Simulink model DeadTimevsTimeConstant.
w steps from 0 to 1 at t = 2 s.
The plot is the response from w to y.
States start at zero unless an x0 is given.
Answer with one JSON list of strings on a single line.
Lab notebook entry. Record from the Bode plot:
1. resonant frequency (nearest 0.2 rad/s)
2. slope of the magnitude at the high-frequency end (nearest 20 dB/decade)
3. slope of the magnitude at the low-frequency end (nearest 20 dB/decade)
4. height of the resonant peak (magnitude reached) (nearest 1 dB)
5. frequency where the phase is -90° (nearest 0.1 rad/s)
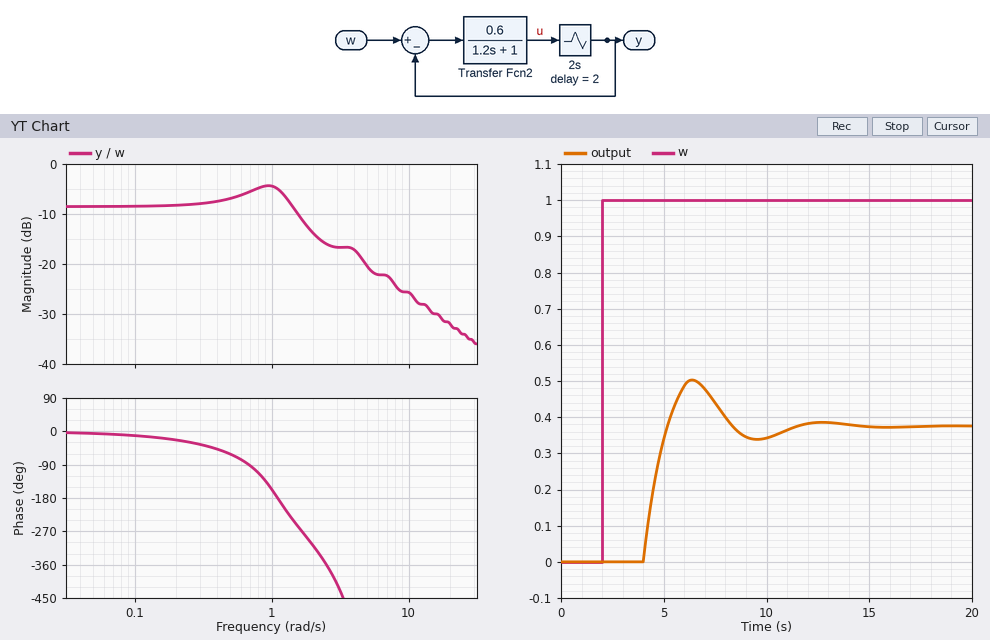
["1.0 rad/s", "-20 dB/decade", "0 dB/decade", "-4 dB", "0.7 rad/s"]
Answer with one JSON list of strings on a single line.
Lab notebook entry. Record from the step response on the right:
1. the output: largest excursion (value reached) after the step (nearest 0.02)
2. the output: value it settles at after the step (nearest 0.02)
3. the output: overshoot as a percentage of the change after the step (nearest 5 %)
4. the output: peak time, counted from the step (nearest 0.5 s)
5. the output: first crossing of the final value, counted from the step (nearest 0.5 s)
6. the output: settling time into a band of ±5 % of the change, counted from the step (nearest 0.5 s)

["0.50", "0.38", "35 %", "4.5 s", "3.0 s", "8.5 s"]
